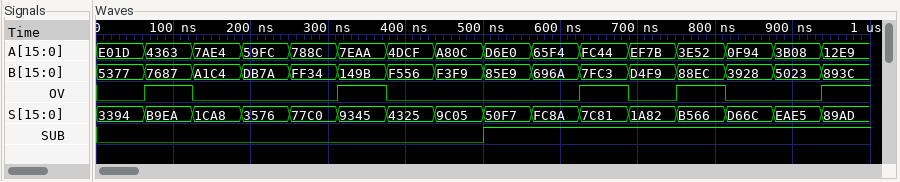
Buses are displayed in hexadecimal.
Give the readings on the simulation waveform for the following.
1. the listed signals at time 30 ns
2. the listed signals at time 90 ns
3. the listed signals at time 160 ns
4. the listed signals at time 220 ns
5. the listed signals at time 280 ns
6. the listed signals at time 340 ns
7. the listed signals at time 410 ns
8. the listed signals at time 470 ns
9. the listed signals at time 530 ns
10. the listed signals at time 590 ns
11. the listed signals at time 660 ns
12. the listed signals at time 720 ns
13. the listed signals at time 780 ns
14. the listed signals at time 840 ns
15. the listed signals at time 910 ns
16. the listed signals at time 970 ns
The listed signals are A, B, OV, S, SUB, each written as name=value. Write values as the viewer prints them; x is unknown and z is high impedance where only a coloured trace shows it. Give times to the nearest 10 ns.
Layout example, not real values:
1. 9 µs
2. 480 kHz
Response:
1. A=E01D, B=5377, OV=0, S=3394, SUB=0
2. A=4363, B=7687, OV=1, S=B9EA, SUB=0
3. A=7AE4, B=A1C4, OV=0, S=1CA8, SUB=0
4. A=59FC, B=DB7A, OV=0, S=3576, SUB=0
5. A=788C, B=FF34, OV=0, S=77C0, SUB=0
6. A=7EAA, B=149B, OV=1, S=9345, SUB=0
7. A=4DCF, B=F556, OV=0, S=4325, SUB=0
8. A=A80C, B=F3F9, OV=0, S=9C05, SUB=0
9. A=D6E0, B=85E9, OV=0, S=50F7, SUB=1
10. A=65F4, B=696A, OV=0, S=FC8A, SUB=1
11. A=FC44, B=7FC3, OV=1, S=7C81, SUB=1
12. A=EF7B, B=D4F9, OV=0, S=1A82, SUB=1
13. A=3E52, B=88EC, OV=1, S=B566, SUB=1
14. A=0F94, B=3928, OV=0, S=D66C, SUB=1
15. A=3B08, B=5023, OV=0, S=EAE5, SUB=1
16. A=12E9, B=893C, OV=1, S=89AD, SUB=1
